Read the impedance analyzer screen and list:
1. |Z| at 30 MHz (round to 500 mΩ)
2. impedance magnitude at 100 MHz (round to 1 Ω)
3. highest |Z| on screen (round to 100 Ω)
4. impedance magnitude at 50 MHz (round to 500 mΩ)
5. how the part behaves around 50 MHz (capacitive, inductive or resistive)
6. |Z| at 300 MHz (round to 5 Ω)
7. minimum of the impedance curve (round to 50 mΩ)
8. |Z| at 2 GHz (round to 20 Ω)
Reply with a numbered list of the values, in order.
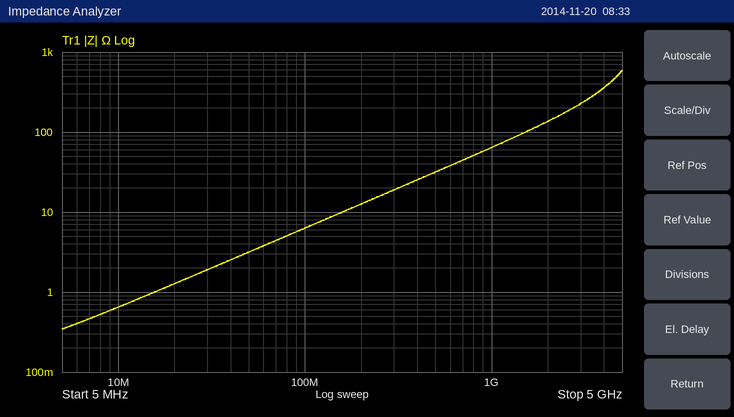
1. 2.0 Ω
2. 6 Ω
3. 600 Ω
4. 3.0 Ω
5. inductive
6. 20 Ω
7. 350 mΩ
8. 140 Ω
